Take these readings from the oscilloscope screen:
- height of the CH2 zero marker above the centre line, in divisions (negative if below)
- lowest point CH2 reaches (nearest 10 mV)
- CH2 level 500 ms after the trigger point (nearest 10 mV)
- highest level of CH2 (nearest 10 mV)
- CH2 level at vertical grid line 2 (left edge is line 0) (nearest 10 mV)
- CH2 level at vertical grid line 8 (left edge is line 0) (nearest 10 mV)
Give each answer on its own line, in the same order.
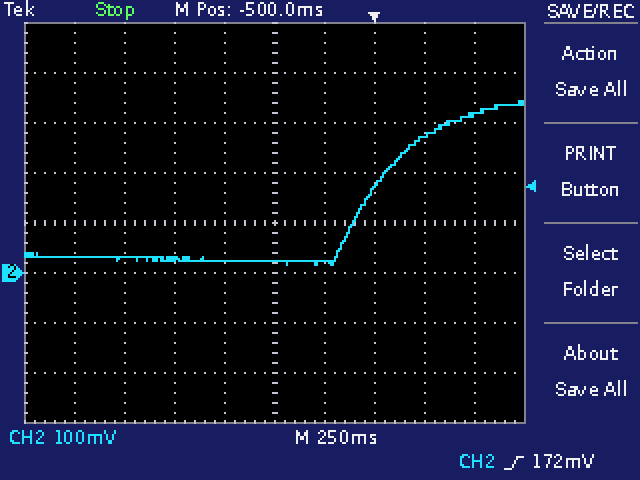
-1.0 div
20 mV
320 mV
340 mV
30 mV
280 mV
